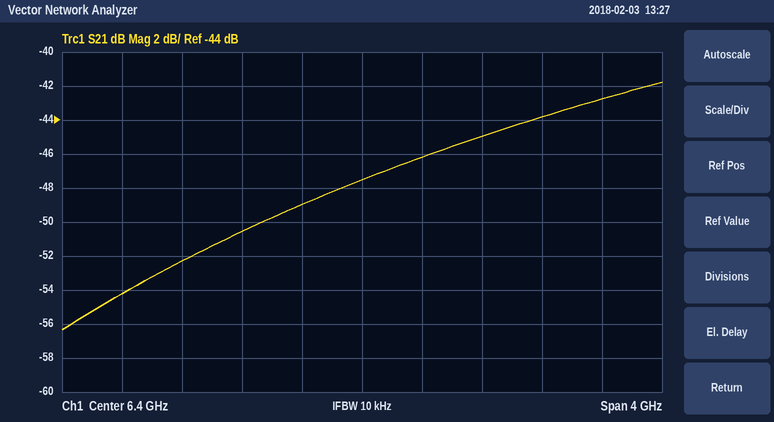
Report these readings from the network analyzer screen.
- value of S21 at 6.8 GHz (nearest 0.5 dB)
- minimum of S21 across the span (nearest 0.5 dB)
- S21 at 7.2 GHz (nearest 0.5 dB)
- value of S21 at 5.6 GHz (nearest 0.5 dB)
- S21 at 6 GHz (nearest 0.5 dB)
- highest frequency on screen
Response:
-46.0 dB
-56.5 dB
-45.0 dB
-50.5 dB
-49.0 dB
8.4 GHz
